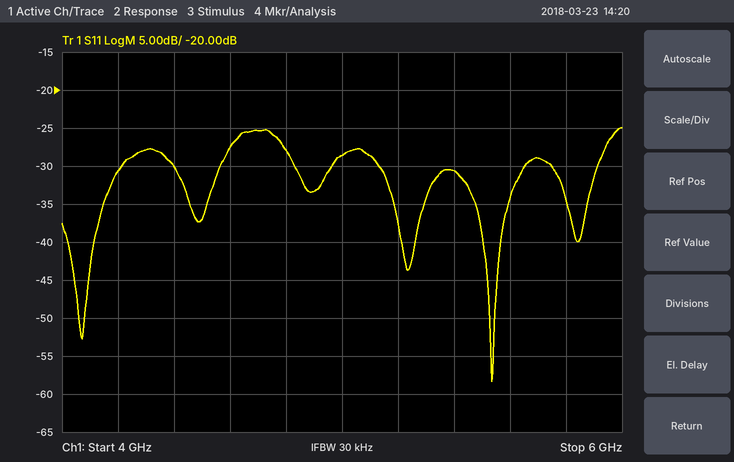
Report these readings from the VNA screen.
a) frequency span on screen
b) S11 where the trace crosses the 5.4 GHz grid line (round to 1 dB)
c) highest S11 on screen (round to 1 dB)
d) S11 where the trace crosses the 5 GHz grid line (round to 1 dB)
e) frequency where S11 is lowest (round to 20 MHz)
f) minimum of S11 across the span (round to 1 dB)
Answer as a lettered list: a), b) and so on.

a) 2 GHz
b) -31 dB
c) -25 dB
d) -29 dB
e) 5.54 GHz
f) -58 dB
